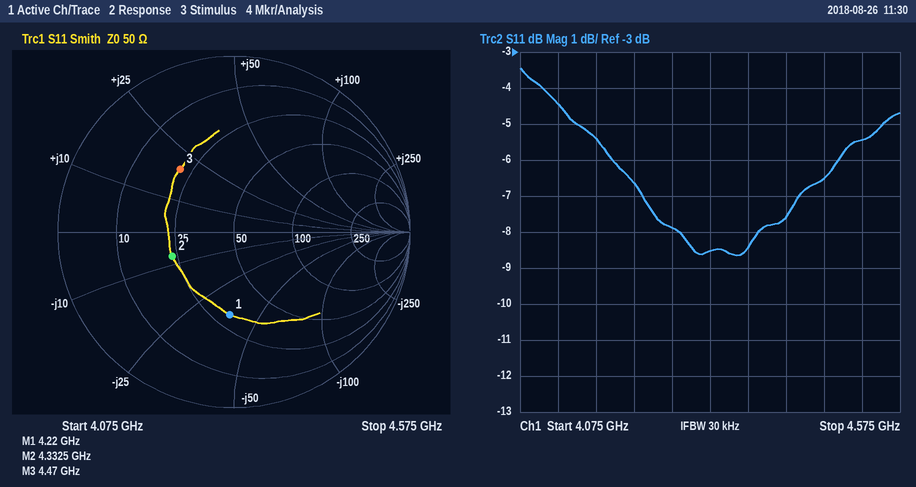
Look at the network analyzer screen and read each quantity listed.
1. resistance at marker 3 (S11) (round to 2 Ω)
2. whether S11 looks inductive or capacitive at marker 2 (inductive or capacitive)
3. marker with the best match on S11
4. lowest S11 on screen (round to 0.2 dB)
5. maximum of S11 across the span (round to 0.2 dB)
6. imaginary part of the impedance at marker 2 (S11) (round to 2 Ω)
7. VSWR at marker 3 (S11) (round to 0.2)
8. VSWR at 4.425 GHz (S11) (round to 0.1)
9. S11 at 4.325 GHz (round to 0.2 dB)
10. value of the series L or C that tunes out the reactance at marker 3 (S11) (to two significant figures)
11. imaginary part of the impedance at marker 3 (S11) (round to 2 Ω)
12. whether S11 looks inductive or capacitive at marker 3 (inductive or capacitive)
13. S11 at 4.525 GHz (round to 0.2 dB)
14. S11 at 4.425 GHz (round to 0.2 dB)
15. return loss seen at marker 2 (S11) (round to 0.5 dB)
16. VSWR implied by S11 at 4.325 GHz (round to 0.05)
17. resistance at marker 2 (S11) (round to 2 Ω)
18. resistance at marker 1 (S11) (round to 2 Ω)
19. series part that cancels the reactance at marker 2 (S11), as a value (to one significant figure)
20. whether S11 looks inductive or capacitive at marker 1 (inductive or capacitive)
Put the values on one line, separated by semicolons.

22 Ω; capacitive; marker 2; -8.6 dB; -3.4 dB; -8 Ω; 2.8; 2.4; -8.6 dB; 1.8 pF; +20 Ω; inductive; -5.4 dB; -7.6 dB; 8.5 dB; 2.20; 24 Ω; 30 Ω; 300 pH; capacitive
